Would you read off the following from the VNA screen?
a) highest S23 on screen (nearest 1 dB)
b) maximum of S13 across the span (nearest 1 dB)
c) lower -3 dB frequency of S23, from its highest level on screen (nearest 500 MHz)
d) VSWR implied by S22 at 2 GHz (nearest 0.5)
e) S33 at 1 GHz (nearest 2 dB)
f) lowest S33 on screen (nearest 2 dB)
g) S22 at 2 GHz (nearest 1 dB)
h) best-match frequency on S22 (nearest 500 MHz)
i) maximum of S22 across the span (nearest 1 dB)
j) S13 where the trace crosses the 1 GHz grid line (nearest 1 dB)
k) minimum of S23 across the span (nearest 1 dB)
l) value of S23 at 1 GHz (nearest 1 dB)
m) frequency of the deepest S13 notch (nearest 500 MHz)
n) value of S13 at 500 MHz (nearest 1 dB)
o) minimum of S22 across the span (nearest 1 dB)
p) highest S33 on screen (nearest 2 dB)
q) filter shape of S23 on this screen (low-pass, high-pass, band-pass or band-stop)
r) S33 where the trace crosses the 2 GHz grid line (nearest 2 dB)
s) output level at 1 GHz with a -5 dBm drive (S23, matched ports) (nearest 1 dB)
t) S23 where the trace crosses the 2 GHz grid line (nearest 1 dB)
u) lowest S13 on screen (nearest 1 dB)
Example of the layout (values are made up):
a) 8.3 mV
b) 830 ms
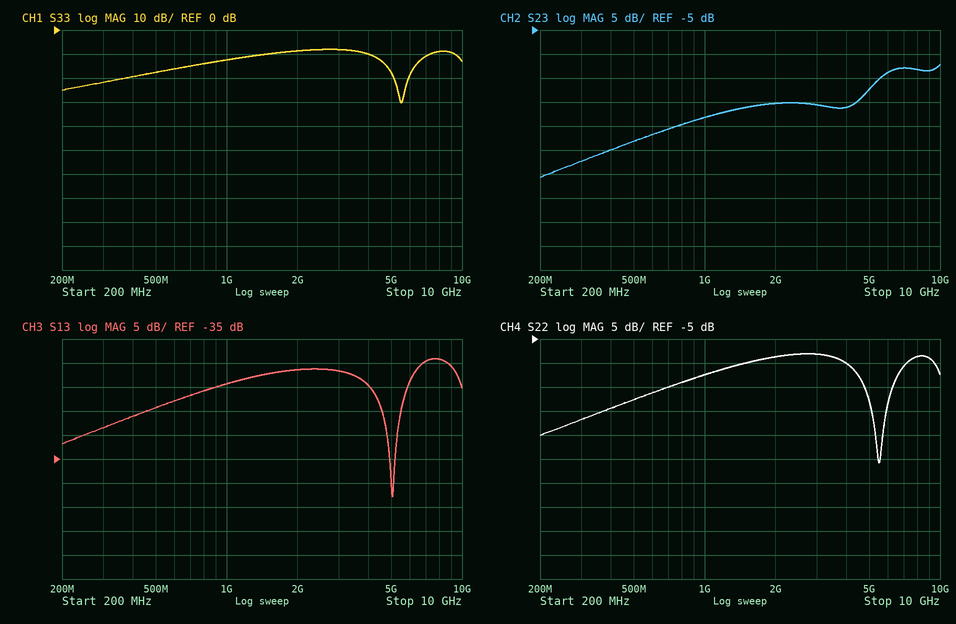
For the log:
a) -12 dB
b) -14 dB
c) 5.5 GHz
d) 2.0
e) -12 dB
f) -30 dB
g) -9 dB
h) 5.5 GHz
i) -8 dB
j) -19 dB
k) -36 dB
l) -23 dB
m) 5.0 GHz
n) -24 dB
o) -31 dB
p) -8 dB
q) high-pass
r) -8 dB
s) -28 dBm
t) -20 dB
u) -43 dB
